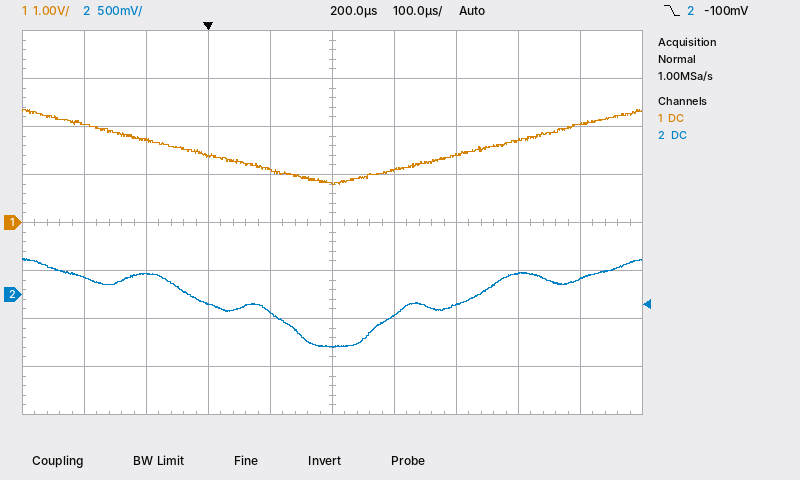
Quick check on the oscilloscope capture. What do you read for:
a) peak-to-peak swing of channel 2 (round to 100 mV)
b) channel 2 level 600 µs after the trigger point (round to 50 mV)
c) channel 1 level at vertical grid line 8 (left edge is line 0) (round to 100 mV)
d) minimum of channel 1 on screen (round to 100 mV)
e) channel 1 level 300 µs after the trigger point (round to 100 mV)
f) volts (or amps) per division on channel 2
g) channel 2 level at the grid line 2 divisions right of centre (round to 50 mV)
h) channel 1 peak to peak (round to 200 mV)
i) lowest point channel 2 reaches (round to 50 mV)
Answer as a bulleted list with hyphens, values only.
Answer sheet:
- 900 mV
- 150 mV
- 1.7 V
- 800 mV
- 1.1 V
- 500 mV
- -100 mV
- 1.6 V
- -550 mV
